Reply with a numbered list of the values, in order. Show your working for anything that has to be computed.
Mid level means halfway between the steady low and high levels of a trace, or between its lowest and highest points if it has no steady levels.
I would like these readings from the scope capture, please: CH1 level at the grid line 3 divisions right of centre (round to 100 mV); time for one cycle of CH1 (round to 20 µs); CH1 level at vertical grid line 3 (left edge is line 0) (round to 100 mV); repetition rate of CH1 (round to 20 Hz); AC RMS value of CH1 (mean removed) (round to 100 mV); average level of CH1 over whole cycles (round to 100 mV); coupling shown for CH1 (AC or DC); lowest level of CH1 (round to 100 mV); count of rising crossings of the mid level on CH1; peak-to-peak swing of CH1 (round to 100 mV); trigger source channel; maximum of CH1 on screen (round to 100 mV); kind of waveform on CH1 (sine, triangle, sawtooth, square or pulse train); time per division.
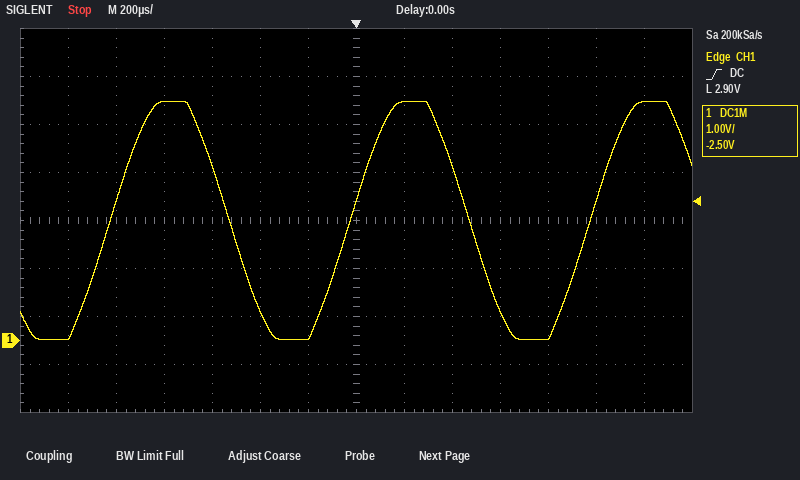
1. 600 mV
2. 1.00 ms
3. 5.0 V
4. 1 / 1.00 ms ≈ 1.00 kHz
5. 5.0 V / (2√2) ≈ 1.8 V
6. (5.0 V + (0.0 V)) / 2 ≈ 2.5 V
7. DC
8. 0.0 V
9. 3
10. 5.0 V − (0.0 V) = 5.0 V
11. CH1
12. 5.0 V
13. sine
14. 200 µs
